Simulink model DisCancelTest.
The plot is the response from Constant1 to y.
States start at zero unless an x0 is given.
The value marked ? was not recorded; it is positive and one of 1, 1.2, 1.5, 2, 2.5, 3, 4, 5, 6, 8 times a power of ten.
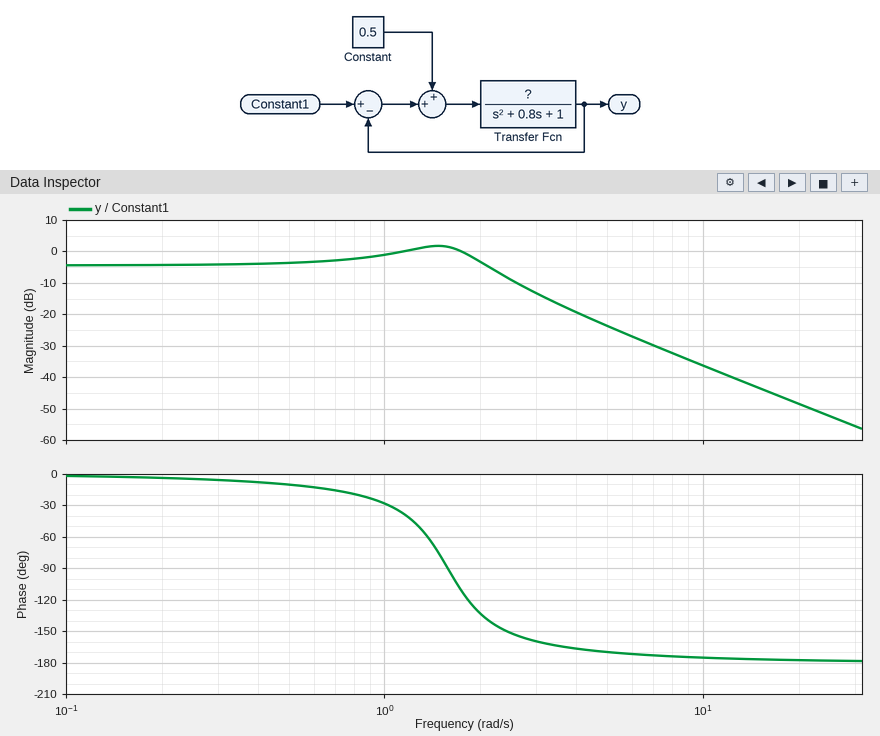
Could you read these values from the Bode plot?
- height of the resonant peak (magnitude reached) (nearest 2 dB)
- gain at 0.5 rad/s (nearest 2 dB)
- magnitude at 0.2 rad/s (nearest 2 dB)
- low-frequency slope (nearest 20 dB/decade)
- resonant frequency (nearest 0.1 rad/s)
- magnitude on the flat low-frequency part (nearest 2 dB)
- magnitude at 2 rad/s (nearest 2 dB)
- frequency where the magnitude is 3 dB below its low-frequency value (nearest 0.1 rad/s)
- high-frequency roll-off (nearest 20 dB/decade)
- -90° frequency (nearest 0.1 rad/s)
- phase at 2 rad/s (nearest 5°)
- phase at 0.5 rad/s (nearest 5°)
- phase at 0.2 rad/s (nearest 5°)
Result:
2 dB
-4 dB
-4 dB
0 dB/decade
1.5 rad/s
-4 dB
-4 dB
2.3 rad/s
-40 dB/decade
1.6 rad/s
-135°
-10°
-5°
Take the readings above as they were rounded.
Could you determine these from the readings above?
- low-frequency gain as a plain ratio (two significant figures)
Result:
0.63
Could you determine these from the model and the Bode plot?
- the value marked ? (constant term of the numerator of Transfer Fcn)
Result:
1.5
